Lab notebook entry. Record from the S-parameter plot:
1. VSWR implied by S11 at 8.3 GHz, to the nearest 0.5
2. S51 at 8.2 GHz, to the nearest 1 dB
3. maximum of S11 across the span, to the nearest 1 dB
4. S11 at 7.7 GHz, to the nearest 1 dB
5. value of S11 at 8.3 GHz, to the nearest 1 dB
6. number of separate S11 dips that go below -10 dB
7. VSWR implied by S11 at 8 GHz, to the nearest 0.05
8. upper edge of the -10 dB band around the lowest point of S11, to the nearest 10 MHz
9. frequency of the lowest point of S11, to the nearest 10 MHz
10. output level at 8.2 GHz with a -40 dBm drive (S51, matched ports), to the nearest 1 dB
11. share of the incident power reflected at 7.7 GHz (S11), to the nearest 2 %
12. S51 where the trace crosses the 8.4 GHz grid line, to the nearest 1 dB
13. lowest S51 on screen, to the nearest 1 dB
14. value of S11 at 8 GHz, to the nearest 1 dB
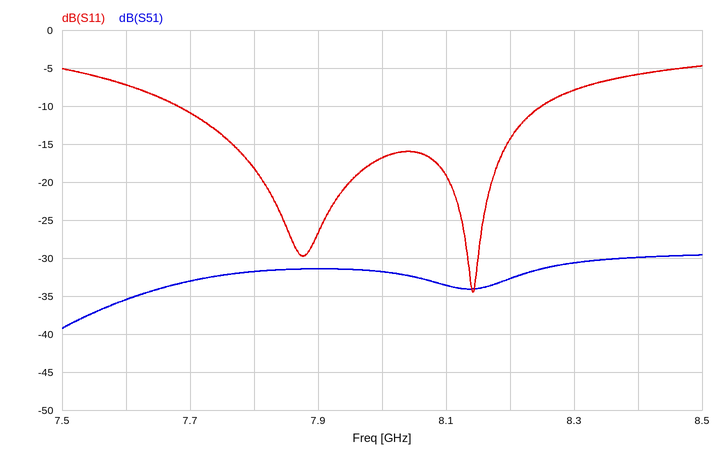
2.5
-33 dB
-5 dB
-11 dB
-8 dB
2
1.35
8.25 GHz
8.14 GHz
-73 dBm
8 %
-30 dB
-39 dB
-17 dB
